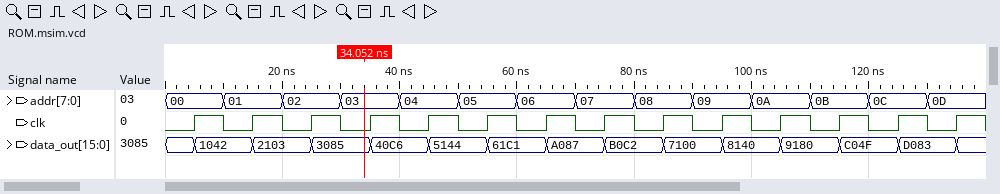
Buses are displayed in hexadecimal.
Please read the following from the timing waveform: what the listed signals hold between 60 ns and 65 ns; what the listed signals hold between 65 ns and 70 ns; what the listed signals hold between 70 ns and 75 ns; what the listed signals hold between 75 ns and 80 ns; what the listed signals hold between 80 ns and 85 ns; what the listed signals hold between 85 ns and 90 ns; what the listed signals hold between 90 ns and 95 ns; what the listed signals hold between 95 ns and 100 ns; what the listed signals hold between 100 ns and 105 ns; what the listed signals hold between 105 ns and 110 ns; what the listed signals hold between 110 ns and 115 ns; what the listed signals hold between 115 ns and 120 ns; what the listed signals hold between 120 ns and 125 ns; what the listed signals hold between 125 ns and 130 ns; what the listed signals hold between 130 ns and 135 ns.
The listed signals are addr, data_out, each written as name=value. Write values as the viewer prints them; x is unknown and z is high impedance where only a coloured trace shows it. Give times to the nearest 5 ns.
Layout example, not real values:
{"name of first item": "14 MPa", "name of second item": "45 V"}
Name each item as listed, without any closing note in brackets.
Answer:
{"what the listed signals hold between 60 ns and 65 ns": "addr=06, data_out=61C1", "what the listed signals hold between 65 ns and 70 ns": "addr=06, data_out=A087", "what the listed signals hold between 70 ns and 75 ns": "addr=07, data_out=A087", "what the listed signals hold between 75 ns and 80 ns": "addr=07, data_out=B0C2", "what the listed signals hold between 80 ns and 85 ns": "addr=08, data_out=B0C2", "what the listed signals hold between 85 ns and 90 ns": "addr=08, data_out=7100", "what the listed signals hold between 90 ns and 95 ns": "addr=09, data_out=7100", "what the listed signals hold between 95 ns and 100 ns": "addr=09, data_out=8140", "what the listed signals hold between 100 ns and 105 ns": "addr=0A, data_out=8140", "what the listed signals hold between 105 ns and 110 ns": "addr=0A, data_out=9180", "what the listed signals hold between 110 ns and 115 ns": "addr=0B, data_out=9180", "what the listed signals hold between 115 ns and 120 ns": "addr=0B, data_out=C04F", "what the listed signals hold between 120 ns and 125 ns": "addr=0C, data_out=C04F", "what the listed signals hold between 125 ns and 130 ns": "addr=0C, data_out=D083", "what the listed signals hold between 130 ns and 135 ns": "addr=0D, data_out=D083"}
